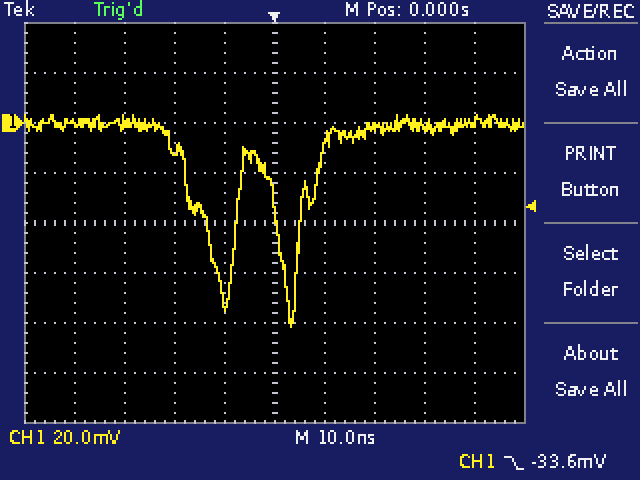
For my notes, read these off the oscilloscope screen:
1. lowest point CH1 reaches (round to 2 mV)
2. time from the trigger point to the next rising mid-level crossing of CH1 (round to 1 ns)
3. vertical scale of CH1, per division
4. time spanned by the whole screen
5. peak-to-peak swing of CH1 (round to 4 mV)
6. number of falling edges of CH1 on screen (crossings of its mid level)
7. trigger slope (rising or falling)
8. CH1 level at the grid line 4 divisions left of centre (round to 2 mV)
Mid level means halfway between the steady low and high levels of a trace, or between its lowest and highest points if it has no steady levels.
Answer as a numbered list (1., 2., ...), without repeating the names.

1. -82 mV
2. 5 ns
3. 20 mV
4. 100 ns
5. 84 mV
6. 2
7. falling
8. 0 mV
